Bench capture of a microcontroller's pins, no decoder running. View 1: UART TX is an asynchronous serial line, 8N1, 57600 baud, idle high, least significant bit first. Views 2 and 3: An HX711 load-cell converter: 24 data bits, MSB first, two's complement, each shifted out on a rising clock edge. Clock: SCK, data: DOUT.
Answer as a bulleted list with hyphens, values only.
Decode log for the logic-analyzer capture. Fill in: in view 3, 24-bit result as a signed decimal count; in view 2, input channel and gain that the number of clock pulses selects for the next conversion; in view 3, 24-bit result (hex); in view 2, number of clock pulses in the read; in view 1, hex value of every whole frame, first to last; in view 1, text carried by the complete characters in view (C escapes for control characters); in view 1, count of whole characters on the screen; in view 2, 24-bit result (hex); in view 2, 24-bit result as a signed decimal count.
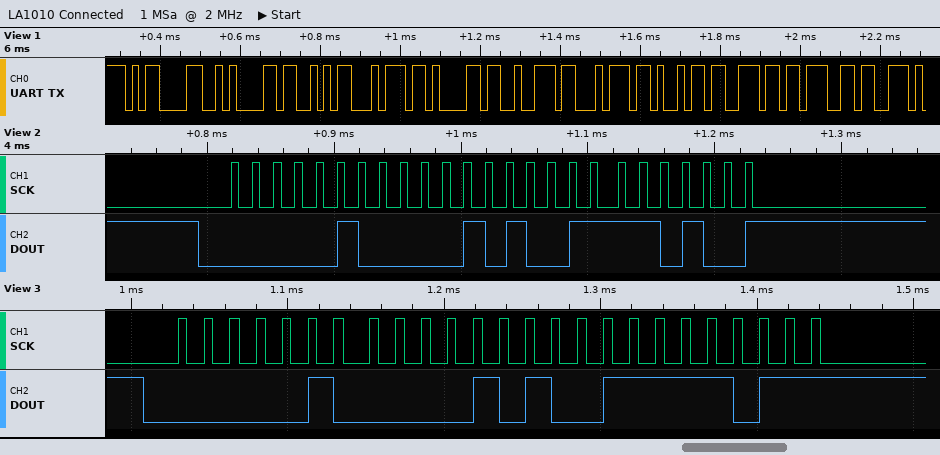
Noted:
- 267515
- channel A, gain 128
- 0x0414FB
- 25
- 0D 0A 53 74 61 72 74 69 6E 67
- "\r\nStarting"
- 10
- 0x0414F4
- 267508
